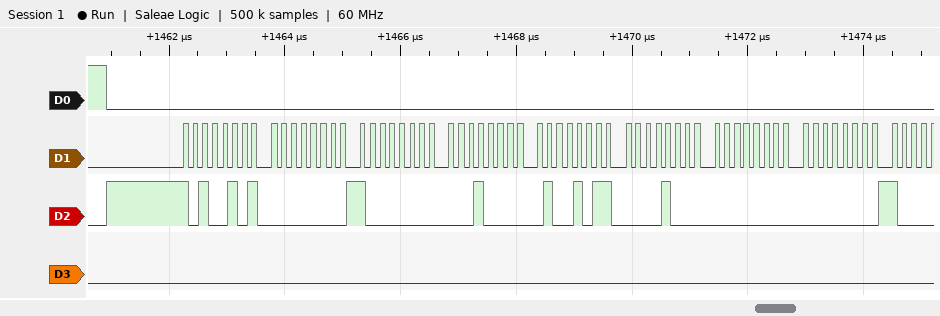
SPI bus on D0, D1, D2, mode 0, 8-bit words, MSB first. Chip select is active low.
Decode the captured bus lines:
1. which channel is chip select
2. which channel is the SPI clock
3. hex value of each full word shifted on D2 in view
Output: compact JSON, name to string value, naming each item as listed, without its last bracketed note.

{"which channel is chip select": "D0", "which channel is the SPI clock": "D1", "hex value of each full word shifted on D2 in view": "A5, 00, 80, 10, 4B, 08, 00, 00"}
